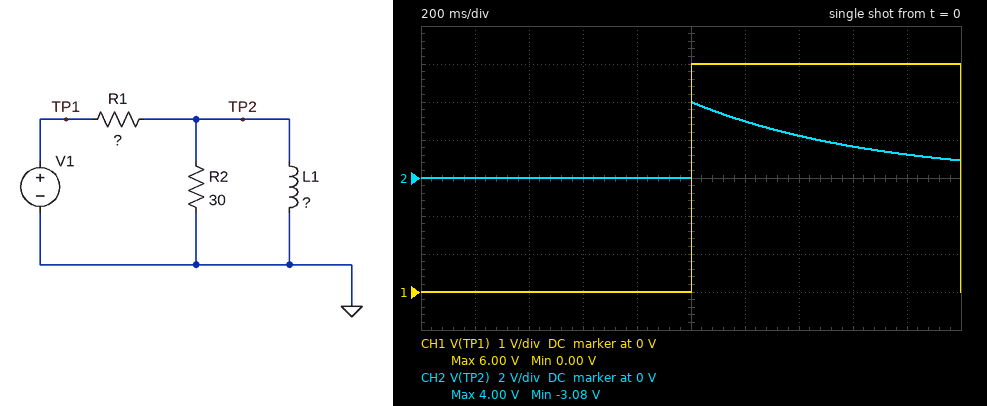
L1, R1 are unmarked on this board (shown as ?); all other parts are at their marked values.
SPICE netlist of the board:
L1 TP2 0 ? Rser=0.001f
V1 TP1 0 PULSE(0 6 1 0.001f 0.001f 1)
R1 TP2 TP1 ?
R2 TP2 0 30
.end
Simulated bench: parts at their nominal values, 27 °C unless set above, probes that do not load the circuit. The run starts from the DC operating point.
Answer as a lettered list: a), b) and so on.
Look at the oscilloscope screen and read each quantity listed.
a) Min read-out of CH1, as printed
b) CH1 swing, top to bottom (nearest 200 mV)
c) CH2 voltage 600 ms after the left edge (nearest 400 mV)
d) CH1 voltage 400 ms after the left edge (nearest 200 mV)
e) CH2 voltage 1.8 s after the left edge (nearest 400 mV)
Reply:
a) 0.00 V
b) 6.0 V
c) 0 V
d) 0 V
e) 1.2 V
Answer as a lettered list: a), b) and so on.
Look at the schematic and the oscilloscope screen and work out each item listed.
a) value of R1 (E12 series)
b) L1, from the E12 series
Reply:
a) 15 Ω
b) 6.8 H
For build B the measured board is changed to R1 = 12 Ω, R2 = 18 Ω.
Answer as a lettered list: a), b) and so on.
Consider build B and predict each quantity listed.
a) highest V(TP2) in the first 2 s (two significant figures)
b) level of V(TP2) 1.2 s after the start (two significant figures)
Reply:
a) 3.6 V
b) 2.9 V
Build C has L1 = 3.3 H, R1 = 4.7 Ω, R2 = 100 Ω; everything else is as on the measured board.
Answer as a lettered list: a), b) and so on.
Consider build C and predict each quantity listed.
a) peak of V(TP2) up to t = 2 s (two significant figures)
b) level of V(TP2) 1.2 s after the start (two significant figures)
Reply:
a) 5.7 V
b) 4.4 V
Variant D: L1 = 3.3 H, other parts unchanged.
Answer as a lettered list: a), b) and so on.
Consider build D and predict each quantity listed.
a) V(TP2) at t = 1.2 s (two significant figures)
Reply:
a) 2.2 V
